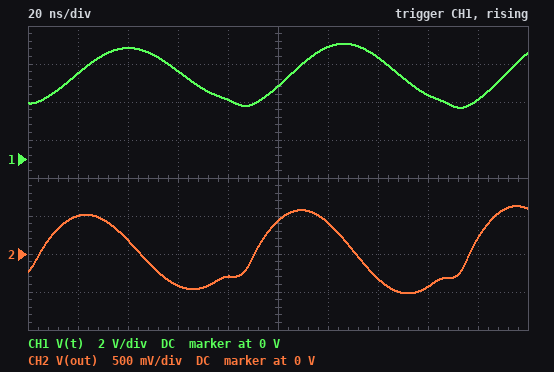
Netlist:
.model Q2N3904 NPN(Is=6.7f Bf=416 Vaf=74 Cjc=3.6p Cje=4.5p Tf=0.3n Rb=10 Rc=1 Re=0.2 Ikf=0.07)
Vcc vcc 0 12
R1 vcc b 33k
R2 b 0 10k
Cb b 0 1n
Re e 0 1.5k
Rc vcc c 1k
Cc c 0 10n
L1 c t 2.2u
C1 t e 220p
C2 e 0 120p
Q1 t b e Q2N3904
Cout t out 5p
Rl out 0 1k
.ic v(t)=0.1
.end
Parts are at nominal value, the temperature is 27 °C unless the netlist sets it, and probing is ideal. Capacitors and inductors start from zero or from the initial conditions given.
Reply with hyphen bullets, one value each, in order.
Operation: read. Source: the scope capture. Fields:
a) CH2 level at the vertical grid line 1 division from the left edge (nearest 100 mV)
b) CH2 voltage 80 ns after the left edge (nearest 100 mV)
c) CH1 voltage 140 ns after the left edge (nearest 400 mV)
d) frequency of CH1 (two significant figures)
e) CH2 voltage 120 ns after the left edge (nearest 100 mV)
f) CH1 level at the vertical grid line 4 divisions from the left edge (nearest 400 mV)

- 500 mV
- -300 mV
- 5.2 V
- 12 MHz
- 400 mV
- 3.2 V
